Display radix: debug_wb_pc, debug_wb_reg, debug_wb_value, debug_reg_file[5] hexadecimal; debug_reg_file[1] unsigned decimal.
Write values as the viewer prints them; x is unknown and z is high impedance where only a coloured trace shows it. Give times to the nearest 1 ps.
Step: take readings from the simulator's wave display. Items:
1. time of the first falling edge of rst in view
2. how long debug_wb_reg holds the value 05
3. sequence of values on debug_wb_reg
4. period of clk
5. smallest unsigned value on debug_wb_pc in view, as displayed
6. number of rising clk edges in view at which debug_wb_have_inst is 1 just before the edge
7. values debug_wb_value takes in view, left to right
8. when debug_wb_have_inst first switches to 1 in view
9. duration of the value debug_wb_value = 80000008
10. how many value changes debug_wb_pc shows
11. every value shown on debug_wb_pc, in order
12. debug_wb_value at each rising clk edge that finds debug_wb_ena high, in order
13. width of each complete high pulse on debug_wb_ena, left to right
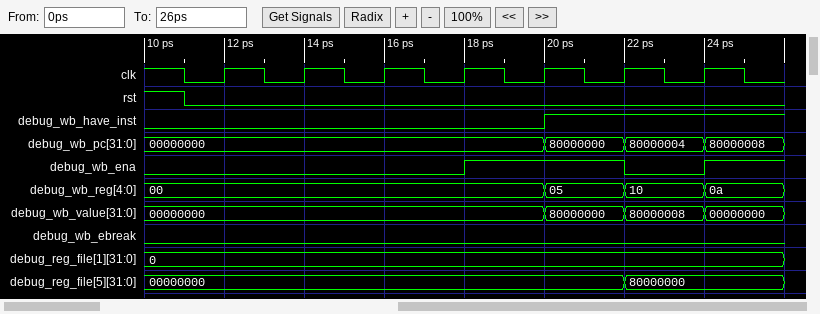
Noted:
11 ps
2 ps
00, 05, 10, 0a
2 ps
00000000
2
00000000, 80000000, 80000008, 00000000
20 ps
2 ps
3
00000000, 80000000, 80000004, 80000008
00000000, 80000000
4 ps
